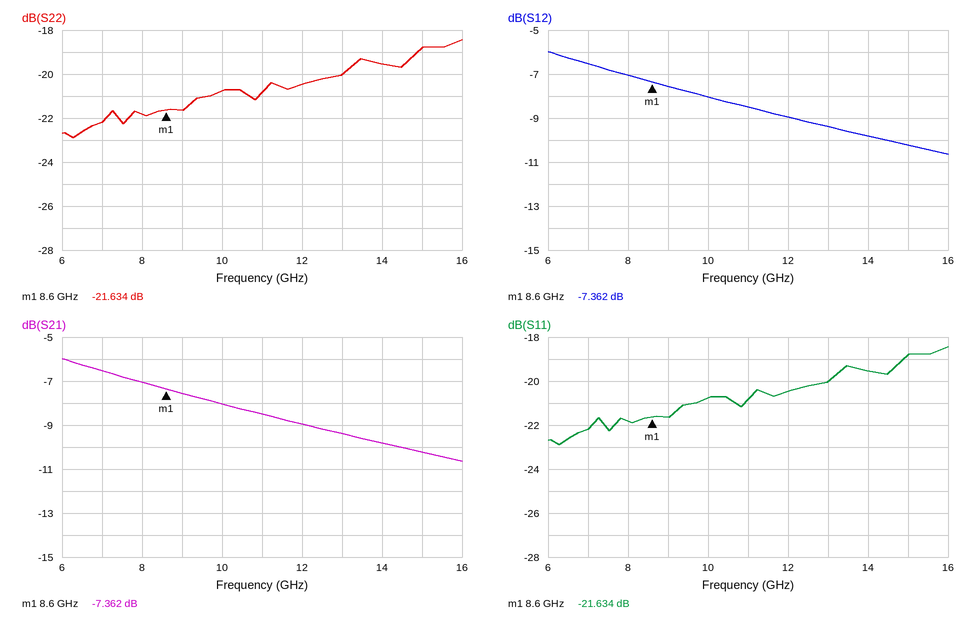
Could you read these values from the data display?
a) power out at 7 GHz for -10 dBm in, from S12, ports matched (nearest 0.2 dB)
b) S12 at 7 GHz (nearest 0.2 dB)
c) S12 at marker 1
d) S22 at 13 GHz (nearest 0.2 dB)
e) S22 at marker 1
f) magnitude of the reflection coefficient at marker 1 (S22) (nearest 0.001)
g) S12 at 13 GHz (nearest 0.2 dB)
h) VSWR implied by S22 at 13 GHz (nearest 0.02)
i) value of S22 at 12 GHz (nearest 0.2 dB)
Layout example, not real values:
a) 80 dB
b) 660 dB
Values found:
a) -16.6 dBm
b) -6.6 dB
c) -7.362 dB
d) -20.0 dB
e) -21.634 dB
f) 0.083
g) -9.4 dB
h) 1.22
i) -20.4 dB
